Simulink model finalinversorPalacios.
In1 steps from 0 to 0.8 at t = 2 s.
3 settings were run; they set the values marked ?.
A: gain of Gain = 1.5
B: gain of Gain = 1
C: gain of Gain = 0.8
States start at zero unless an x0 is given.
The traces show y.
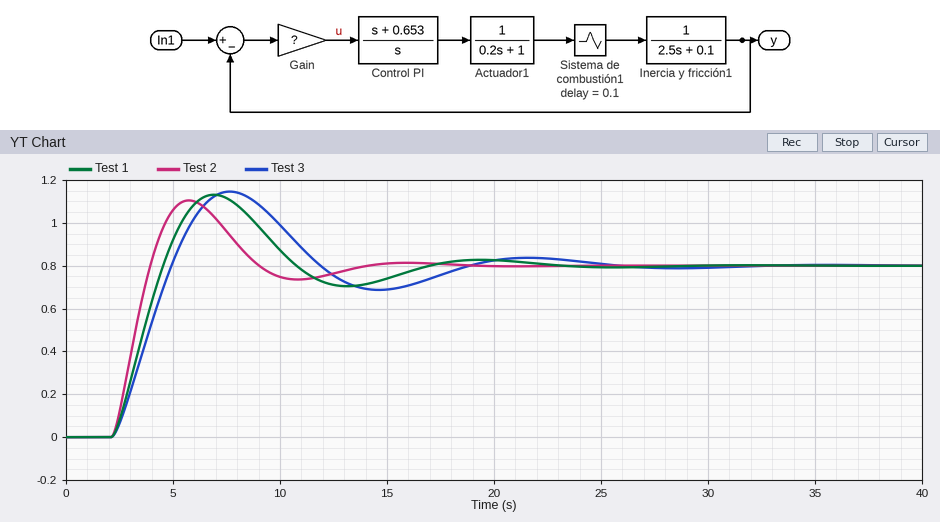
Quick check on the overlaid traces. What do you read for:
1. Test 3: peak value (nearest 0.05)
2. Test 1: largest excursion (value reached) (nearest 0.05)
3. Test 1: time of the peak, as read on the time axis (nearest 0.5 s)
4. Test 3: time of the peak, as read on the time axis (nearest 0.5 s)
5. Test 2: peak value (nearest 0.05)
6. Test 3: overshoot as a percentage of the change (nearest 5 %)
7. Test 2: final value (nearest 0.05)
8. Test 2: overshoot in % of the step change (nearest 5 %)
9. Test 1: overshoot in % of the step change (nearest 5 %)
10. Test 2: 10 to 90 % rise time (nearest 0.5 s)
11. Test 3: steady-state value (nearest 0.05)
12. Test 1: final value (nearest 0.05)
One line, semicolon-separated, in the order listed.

1.15; 1.15; 7.0 s; 7.5 s; 1.10; 45 %; 0.80; 40 %; 40 %; 1.5 s; 0.80; 0.80
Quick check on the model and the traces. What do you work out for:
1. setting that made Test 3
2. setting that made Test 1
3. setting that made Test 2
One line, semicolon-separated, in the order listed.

C; B; A
